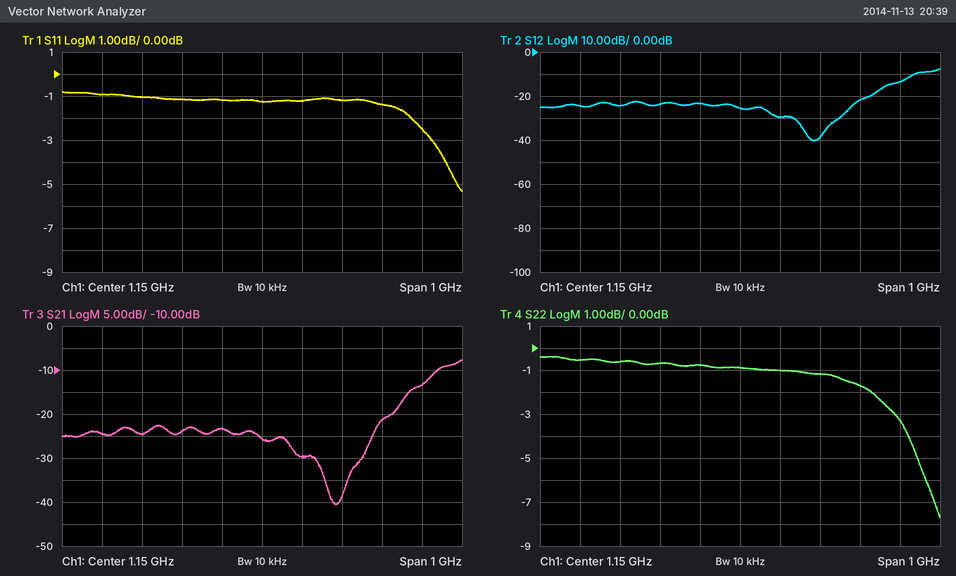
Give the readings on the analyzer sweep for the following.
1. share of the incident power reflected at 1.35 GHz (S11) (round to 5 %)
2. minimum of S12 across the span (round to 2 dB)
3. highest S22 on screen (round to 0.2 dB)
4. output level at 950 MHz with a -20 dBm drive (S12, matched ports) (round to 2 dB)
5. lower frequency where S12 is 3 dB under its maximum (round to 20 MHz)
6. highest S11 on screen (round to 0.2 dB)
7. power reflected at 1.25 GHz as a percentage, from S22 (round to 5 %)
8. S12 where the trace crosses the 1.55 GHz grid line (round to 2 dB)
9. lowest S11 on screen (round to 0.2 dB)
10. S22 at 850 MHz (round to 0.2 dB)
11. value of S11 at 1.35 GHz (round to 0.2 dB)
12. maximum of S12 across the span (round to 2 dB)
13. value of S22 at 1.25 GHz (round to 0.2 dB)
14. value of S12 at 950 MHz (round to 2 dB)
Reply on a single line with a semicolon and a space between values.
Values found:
75 %; -40 dB; -0.4 dB; -44 dBm; 1.58 GHz; -0.8 dB; 80 %; -14 dB; -5.4 dB; -0.6 dB; -1.2 dB; -8 dB; -1.0 dB; -24 dB
